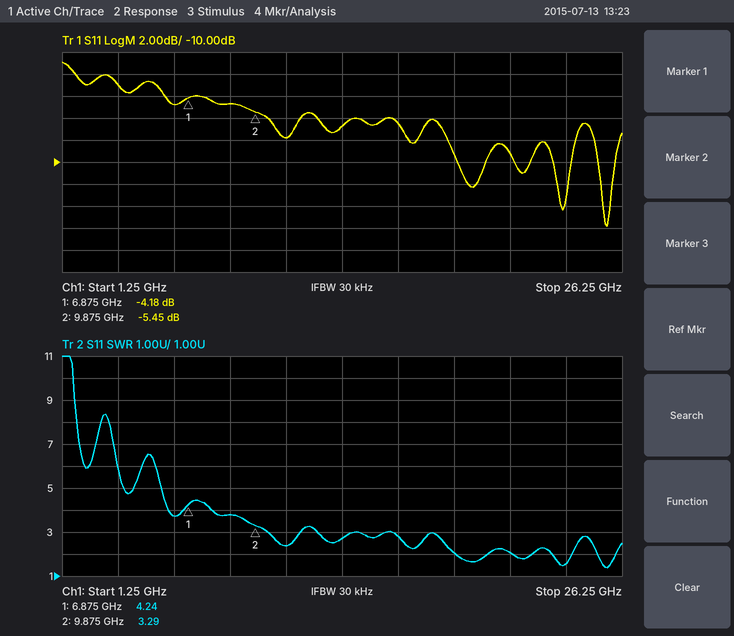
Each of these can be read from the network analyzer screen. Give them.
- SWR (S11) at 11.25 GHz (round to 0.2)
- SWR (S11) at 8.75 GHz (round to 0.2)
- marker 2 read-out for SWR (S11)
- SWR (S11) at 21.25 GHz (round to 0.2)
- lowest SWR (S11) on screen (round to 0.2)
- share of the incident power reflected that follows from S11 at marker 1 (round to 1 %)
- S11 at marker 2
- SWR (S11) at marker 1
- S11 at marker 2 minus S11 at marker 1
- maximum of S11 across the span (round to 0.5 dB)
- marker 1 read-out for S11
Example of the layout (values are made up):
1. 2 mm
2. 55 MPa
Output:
1. 2.4
2. 3.8
3. 3.29
4. 2.0
5. 1.4
6. 38 %
7. -5.45 dB
8. 4.24
9. -1.27 dB
10. -1.0 dB
11. -4.18 dB
